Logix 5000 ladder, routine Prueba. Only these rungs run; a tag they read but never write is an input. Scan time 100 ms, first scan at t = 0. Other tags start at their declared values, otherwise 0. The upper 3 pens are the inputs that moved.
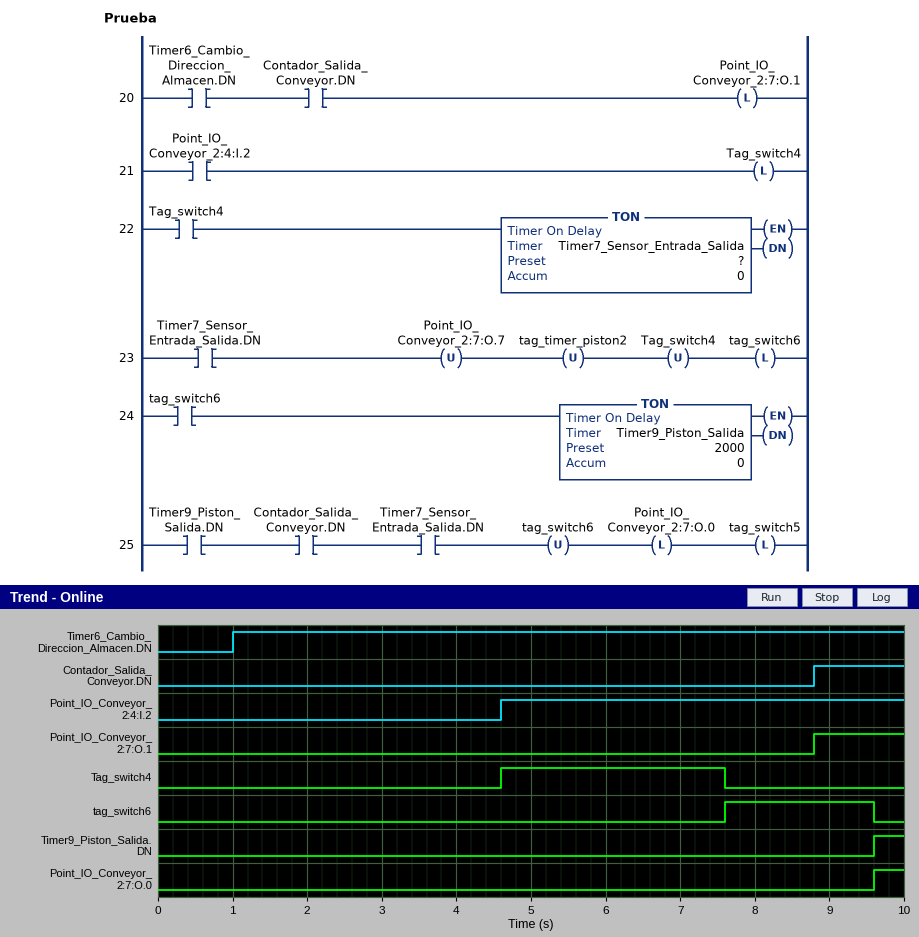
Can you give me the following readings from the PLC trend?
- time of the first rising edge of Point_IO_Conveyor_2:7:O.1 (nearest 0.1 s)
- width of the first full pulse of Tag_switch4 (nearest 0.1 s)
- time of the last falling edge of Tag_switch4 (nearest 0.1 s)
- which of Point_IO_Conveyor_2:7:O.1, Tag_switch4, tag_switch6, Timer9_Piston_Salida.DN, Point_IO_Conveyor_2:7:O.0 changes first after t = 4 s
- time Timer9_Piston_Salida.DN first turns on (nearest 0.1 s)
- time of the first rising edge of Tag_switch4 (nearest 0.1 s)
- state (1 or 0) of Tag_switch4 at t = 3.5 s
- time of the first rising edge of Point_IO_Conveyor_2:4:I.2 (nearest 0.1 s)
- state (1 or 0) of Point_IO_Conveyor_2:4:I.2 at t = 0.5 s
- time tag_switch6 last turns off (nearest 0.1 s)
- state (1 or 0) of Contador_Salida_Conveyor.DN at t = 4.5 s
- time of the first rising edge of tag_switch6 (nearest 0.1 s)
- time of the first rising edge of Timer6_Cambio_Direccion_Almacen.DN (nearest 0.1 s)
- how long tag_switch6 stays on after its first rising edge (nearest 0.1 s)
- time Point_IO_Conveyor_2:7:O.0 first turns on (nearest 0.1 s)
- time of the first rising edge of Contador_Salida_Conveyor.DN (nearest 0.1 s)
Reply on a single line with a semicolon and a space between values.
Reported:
8.8 s; 3.0 s; 7.6 s; Tag_switch4; 9.6 s; 4.6 s; 0; 4.6 s; 0; 9.6 s; 0; 7.6 s; 1.0 s; 2.0 s; 9.6 s; 8.8 s
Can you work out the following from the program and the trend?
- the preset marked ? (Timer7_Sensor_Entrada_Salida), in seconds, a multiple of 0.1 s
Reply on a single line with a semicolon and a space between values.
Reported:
3.0 s
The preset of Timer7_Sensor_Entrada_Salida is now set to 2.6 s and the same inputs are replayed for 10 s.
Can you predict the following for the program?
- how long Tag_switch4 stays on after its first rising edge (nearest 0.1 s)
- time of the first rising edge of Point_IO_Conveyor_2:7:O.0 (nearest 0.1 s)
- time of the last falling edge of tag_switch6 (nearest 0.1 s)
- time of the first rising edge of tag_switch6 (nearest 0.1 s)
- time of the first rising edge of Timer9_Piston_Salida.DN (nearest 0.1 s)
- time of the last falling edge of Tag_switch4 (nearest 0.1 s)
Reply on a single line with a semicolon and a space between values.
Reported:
2.6 s; 9.2 s; 9.2 s; 7.2 s; 9.2 s; 7.2 s
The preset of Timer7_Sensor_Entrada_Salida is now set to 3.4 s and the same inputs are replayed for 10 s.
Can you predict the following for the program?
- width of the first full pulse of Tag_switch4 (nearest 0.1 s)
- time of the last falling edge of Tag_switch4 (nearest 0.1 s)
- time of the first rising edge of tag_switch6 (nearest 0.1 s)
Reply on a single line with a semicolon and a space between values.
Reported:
3.4 s; 8.0 s; 8.0 s
